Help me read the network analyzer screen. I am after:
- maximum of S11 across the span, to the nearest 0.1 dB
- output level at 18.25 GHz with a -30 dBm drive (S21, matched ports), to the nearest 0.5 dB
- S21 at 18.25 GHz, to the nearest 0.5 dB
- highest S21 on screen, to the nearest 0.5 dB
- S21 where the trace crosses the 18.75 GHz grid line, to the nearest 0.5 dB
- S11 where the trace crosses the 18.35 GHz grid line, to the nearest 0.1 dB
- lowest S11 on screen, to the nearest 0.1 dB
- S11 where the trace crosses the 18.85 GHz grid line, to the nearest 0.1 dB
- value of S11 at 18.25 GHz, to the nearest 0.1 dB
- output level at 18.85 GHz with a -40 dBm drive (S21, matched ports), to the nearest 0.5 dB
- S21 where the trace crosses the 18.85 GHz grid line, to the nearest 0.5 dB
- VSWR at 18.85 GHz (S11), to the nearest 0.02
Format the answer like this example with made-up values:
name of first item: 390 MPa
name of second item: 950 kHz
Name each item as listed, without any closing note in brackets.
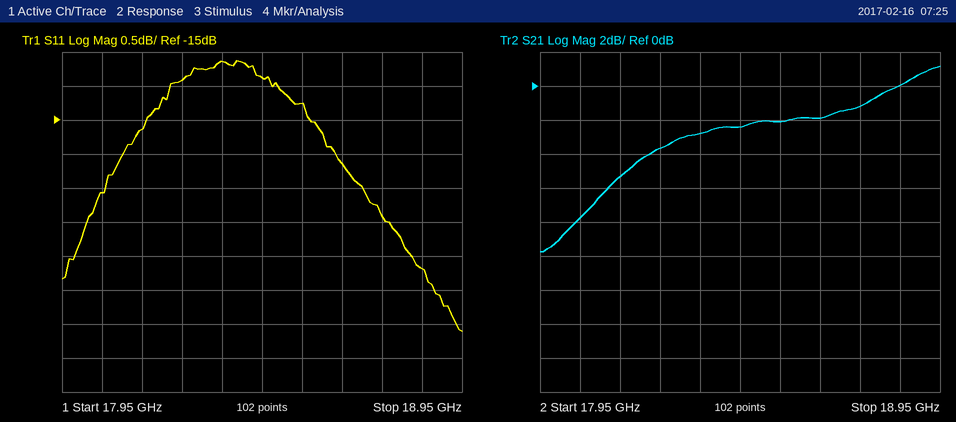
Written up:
maximum of S11 across the span, to the nearest 0.1 dB: -14.1 dB
output level at 18.25 GHz with a -30 dBm drive (S21, matched ports), to the nearest 0.5 dB: -33.5 dBm
S21 at 18.25 GHz, to the nearest 0.5 dB: -3.5 dB
highest S21 on screen, to the nearest 0.5 dB: 1.0 dB
S21 where the trace crosses the 18.75 GHz grid line, to the nearest 0.5 dB: -1.0 dB
S11 where the trace crosses the 18.35 GHz grid line, to the nearest 0.1 dB: -14.1 dB
lowest S11 on screen, to the nearest 0.1 dB: -18.1 dB
S11 where the trace crosses the 18.85 GHz grid line, to the nearest 0.1 dB: -17.2 dB
value of S11 at 18.25 GHz, to the nearest 0.1 dB: -14.4 dB
output level at 18.85 GHz with a -40 dBm drive (S21, matched ports), to the nearest 0.5 dB: -40.0 dBm
S21 where the trace crosses the 18.85 GHz grid line, to the nearest 0.5 dB: 0.0 dB
VSWR at 18.85 GHz (S11), to the nearest 0.02: 1.32
